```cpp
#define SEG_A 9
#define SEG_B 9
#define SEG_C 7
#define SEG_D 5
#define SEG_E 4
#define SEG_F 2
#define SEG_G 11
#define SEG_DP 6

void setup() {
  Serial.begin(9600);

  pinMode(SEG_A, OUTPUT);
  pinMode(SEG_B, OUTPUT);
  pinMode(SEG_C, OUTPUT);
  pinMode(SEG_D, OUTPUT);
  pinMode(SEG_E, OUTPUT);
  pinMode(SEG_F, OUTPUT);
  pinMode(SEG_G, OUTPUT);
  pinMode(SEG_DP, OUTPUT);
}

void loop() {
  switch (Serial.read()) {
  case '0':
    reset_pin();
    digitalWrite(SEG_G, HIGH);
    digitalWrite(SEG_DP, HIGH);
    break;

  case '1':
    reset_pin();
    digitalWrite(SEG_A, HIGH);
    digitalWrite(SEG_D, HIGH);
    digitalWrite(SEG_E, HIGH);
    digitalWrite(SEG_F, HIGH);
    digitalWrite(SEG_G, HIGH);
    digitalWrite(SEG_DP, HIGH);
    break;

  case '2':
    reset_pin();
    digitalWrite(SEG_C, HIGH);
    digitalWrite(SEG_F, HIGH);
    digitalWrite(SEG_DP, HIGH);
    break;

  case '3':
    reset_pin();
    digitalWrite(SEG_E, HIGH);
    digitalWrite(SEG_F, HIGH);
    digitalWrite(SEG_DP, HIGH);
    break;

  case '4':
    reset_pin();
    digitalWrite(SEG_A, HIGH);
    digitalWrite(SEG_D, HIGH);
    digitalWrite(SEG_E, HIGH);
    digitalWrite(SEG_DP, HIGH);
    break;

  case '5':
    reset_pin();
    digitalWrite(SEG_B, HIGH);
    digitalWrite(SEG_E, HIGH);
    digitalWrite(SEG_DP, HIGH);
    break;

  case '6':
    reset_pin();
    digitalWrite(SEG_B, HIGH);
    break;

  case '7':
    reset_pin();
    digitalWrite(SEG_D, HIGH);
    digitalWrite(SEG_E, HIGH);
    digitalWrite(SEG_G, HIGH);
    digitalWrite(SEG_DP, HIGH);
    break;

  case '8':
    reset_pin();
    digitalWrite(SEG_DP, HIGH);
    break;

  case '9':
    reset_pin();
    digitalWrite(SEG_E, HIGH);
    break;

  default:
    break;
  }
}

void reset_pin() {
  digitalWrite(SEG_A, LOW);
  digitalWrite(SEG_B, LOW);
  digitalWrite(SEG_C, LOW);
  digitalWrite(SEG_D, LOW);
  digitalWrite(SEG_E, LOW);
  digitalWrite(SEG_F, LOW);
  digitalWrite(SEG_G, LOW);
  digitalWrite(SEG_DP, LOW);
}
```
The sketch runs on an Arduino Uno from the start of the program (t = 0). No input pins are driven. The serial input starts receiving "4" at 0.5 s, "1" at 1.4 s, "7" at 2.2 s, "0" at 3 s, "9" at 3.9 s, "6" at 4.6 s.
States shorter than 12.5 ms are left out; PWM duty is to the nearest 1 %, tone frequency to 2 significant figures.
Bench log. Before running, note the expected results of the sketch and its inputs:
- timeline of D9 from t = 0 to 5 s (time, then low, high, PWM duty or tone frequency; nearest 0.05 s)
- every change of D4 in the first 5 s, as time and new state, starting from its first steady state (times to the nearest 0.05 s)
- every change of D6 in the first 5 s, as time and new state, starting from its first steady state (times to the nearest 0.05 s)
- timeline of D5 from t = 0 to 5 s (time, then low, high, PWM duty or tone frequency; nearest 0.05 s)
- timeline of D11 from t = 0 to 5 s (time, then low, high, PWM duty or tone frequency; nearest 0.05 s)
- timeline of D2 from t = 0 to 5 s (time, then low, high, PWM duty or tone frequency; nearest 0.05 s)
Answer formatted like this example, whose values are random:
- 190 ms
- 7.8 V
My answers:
- 0 s low; 0.5 s high; 2.2 s low; 4.6 s high
- 0 s low; 0.5 s high; 3 s low; 3.9 s high; 4.6 s low
- 0 s low; 0.5 s high; 3.9 s low
- 0 s low; 0.5 s high; 3 s low
- 0 s low; 1.4 s high; 3.9 s low
- 0 s low; 1.4 s high; 2.2 s low
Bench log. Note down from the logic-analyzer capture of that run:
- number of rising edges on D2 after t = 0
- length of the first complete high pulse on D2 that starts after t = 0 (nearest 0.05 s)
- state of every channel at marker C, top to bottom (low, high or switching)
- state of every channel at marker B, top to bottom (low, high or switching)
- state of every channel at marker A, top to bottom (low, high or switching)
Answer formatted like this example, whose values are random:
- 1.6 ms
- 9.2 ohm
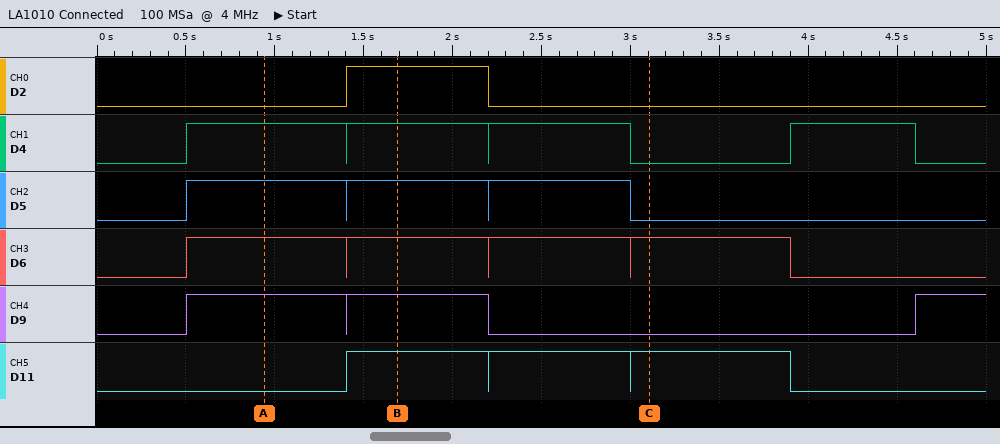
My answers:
- 1
- 0.80 s
- D2 low, D4 low, D5 low, D6 high, D9 low, D11 high
- D2 high, D4 high, D5 high, D6 high, D9 high, D11 high
- D2 low, D4 high, D5 high, D6 high, D9 high, D11 low
